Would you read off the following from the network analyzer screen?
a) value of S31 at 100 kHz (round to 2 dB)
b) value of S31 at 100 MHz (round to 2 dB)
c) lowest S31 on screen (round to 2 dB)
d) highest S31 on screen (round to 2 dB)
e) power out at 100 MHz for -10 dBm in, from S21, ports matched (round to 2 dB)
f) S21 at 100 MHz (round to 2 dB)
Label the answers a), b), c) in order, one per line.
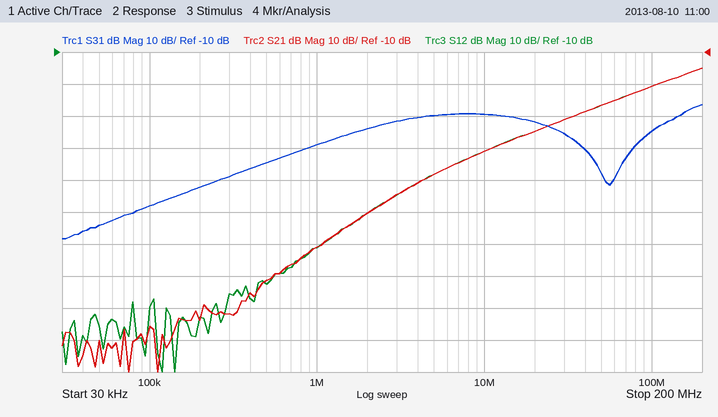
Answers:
a) -58 dB
b) -34 dB
c) -68 dB
d) -26 dB
e) -30 dBm
f) -20 dB
